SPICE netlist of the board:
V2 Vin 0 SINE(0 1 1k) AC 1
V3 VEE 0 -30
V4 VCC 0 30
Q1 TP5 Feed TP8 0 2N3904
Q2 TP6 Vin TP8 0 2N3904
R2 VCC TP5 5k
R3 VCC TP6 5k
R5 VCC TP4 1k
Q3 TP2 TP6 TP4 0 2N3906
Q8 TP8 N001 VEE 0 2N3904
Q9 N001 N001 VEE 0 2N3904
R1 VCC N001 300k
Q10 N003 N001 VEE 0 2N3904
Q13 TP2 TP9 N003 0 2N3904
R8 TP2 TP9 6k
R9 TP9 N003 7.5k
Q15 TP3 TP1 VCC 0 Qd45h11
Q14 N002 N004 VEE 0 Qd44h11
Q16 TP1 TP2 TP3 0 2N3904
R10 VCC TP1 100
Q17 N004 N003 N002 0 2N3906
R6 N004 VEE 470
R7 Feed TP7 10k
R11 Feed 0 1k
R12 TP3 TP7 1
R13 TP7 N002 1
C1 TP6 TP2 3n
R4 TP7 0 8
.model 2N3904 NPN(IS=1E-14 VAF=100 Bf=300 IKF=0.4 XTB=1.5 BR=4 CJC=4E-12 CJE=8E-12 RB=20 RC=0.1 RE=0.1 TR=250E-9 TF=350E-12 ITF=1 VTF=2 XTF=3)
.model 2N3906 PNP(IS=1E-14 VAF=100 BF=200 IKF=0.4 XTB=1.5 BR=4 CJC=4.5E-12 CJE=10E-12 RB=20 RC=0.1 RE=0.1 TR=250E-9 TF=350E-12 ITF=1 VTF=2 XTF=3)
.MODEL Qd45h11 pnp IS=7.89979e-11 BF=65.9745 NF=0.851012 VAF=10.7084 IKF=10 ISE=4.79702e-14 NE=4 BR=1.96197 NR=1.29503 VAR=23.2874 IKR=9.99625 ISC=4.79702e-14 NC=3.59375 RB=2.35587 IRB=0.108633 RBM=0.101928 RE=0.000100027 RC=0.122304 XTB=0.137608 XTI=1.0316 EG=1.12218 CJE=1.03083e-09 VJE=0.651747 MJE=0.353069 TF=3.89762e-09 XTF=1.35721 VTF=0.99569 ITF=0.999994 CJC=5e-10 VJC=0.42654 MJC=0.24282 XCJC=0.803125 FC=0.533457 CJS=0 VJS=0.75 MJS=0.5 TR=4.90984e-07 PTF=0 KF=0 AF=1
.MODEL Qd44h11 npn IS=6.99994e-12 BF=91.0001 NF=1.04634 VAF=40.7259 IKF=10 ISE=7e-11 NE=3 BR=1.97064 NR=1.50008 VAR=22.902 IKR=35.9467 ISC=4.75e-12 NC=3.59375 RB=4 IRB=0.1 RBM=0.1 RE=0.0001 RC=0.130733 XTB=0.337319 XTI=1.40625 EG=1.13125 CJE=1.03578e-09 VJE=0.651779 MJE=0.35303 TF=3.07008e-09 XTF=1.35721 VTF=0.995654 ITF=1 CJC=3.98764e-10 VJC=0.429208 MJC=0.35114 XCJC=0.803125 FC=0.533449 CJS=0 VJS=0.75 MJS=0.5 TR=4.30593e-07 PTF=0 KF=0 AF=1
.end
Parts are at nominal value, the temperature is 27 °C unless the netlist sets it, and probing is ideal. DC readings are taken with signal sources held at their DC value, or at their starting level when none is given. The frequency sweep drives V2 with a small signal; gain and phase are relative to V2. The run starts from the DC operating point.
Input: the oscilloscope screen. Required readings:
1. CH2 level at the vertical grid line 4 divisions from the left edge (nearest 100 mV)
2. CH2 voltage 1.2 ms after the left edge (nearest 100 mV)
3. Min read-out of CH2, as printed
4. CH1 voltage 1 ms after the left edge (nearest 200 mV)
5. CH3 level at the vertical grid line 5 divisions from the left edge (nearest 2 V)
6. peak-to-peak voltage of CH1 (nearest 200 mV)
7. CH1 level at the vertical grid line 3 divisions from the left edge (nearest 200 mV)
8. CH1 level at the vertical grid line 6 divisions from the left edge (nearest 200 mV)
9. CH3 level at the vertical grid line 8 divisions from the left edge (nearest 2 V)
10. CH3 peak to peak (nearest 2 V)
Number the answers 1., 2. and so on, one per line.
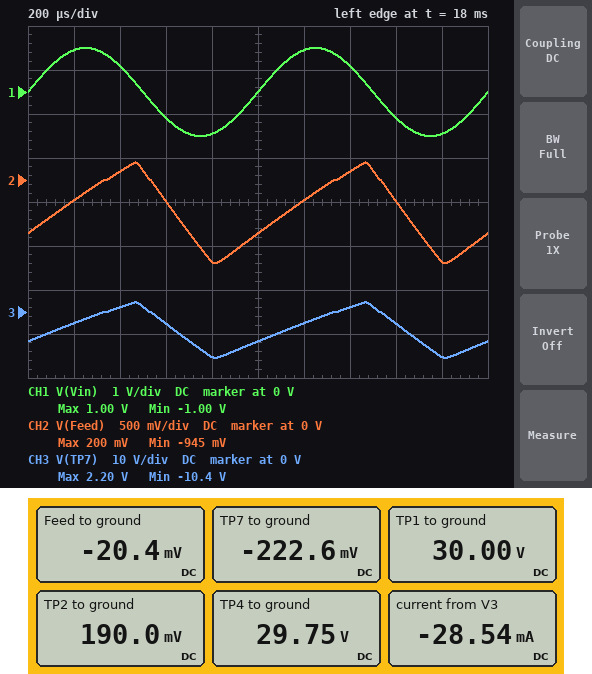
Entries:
1. -900 mV
2. -200 mV
3. -945 mV
4. 0 V
5. -6 V
6. 2.0 V
7. -600 mV
8. 1.0 V
9. -2 V
10. 12 V
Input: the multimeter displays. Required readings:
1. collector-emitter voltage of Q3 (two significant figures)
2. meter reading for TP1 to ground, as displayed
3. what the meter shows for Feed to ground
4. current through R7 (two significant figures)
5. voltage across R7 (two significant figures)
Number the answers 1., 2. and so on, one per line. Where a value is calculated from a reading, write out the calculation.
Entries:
1. 190 mV - 29.75 V = -30 V
2. 30.00 V
3. -20.4 mV
4. (-20.4 mV - (-222.6 mV)) / 10 kΩ = 20 µA
5. -20.4 mV - (-222.6 mV) = 200 mV
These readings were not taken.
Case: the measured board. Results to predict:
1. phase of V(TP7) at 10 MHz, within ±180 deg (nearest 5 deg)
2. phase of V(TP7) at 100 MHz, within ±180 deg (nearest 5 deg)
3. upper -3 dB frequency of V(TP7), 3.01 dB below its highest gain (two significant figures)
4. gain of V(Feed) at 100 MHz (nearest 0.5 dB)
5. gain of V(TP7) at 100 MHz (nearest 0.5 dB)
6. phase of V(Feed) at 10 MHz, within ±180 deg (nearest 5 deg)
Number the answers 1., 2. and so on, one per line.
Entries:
1. 0 deg
2. 50 deg
3. 8.7 kHz
4. -2.0 dB
5. -45.5 dB
6. 30 deg
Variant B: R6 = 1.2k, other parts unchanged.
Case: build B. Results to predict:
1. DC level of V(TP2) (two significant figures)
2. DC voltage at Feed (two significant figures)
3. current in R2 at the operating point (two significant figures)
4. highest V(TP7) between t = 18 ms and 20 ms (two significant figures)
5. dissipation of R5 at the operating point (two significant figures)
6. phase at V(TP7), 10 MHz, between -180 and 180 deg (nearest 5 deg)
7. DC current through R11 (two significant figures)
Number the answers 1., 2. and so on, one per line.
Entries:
1. 210 mV
2. -21 mV
3. 78 µA
4. 2.1 V
5. 63 µW
6. -5 deg
7. 21 µA
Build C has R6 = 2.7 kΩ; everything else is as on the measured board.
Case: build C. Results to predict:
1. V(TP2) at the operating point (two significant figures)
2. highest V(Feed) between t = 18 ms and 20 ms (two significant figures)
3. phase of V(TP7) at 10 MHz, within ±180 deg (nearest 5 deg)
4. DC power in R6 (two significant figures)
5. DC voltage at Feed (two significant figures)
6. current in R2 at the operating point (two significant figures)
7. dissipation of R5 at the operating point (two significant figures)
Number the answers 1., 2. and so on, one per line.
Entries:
1. 220 mV
2. 190 mV
3. -5 deg
4. 130 µW
5. -21 mV
6. 78 µA
7. 63 µW
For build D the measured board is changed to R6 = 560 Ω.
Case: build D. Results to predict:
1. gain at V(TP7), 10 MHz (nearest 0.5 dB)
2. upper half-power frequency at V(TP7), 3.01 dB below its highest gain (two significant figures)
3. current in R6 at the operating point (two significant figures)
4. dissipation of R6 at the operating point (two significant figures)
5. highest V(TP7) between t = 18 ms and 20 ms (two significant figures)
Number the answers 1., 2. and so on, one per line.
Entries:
1. -10.5 dB
2. 8.6 kHz
3. 1.0 mA
4. 610 µW
5. 2.2 V
